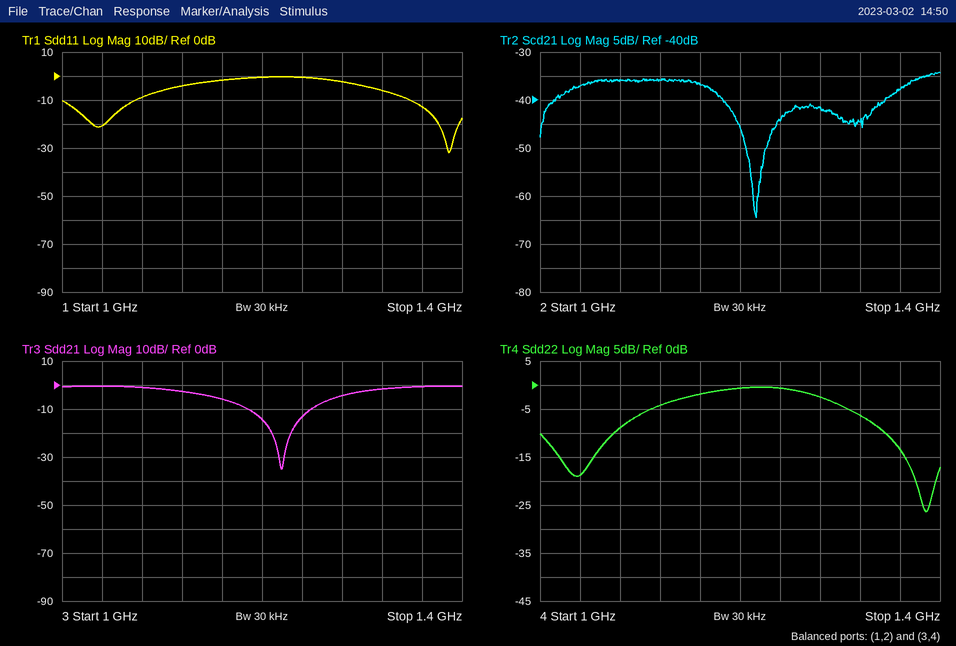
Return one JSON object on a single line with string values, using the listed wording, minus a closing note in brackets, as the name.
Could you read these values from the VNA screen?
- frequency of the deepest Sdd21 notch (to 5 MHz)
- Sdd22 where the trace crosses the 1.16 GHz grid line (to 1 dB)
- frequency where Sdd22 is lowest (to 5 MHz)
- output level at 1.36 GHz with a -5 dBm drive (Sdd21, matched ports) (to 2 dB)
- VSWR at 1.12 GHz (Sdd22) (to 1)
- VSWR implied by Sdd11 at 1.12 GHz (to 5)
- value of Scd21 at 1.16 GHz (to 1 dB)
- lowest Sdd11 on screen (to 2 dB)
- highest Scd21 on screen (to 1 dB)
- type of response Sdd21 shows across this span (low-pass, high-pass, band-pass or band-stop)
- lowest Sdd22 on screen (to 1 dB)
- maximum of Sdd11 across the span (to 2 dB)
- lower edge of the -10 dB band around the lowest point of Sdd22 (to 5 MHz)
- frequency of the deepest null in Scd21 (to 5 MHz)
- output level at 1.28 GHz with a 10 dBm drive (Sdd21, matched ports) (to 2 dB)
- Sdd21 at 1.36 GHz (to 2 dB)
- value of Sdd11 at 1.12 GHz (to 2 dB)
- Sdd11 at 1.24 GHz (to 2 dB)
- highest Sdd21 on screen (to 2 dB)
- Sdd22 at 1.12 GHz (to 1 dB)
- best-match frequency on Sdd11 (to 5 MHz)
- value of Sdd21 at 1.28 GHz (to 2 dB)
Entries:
{"frequency of the deepest Sdd21 notch": "1.220 GHz", "Sdd22 where the trace crosses the 1.16 GHz grid line": "-2 dB", "frequency where Sdd22 is lowest": "1.385 GHz", "output level at 1.36 GHz with a -5 dBm drive (Sdd21, matched ports)": "-6 dBm", "VSWR at 1.12 GHz (Sdd22)": "4", "VSWR implied by Sdd11 at 1.12 GHz": "5", "value of Scd21 at 1.16 GHz": "-37 dB", "lowest Sdd11 on screen": "-32 dB", "highest Scd21 on screen": "-34 dB", "type of response Sdd21 shows across this span": "band-stop", "lowest Sdd22 on screen": "-26 dB", "maximum of Sdd11 across the span": "0 dB", "lower edge of the -10 dB band around the lowest point of Sdd22": "1.345 GHz", "frequency of the deepest null in Scd21": "1.215 GHz", "output level at 1.28 GHz with a 10 dBm drive (Sdd21, matched ports)": "6 dBm", "Sdd21 at 1.36 GHz": "0 dB", "value of Sdd11 at 1.12 GHz": "-4 dB", "Sdd11 at 1.24 GHz": "0 dB", "highest Sdd21 on screen": "0 dB", "Sdd22 at 1.12 GHz": "-4 dB", "best-match frequency on Sdd11": "1.385 GHz", "value of Sdd21 at 1.28 GHz": "-4 dB"}
